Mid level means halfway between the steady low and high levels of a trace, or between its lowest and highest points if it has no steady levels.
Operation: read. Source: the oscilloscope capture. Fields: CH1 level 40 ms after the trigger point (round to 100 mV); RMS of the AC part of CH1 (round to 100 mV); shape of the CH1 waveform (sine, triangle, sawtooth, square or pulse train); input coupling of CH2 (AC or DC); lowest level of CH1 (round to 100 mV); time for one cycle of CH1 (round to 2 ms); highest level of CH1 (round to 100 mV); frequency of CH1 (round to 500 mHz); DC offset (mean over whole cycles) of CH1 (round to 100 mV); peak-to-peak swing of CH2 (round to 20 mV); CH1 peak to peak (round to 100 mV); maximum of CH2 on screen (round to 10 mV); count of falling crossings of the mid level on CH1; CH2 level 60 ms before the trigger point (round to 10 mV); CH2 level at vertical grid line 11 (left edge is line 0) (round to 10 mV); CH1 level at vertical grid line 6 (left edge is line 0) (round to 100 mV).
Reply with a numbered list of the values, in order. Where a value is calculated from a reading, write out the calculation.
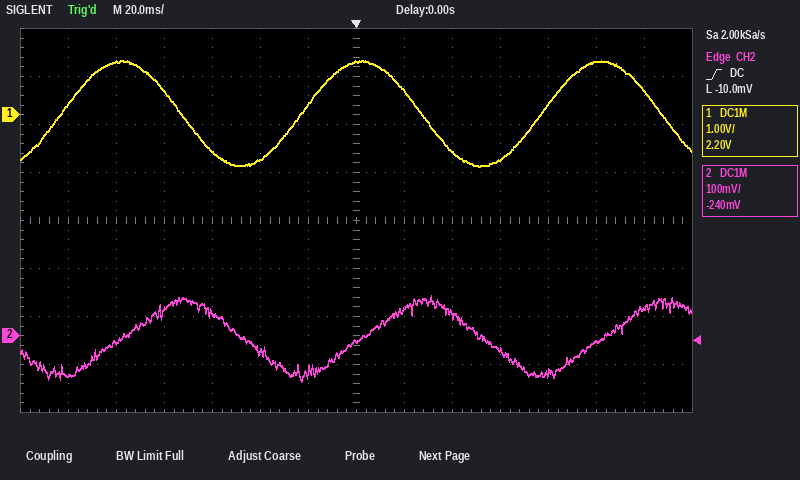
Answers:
1. -800 mV
2. 2.2 V / (2√2) ≈ 778 mV, so 800 mV to the nearest 100 mV
3. sine
4. DC
5. -1.1 V
6. 100 ms
7. 1.1 V
8. 1 / 100 ms ≈ 10.0 Hz
9. (1.1 V + (-1.1 V)) / 2 ≈ 0.0 V
10. 180 mV
11. 1.1 V − (-1.1 V) = 2.2 V
12. 80 mV
13. 3
14. 50 mV
15. -80 mV
16. 200 mV
